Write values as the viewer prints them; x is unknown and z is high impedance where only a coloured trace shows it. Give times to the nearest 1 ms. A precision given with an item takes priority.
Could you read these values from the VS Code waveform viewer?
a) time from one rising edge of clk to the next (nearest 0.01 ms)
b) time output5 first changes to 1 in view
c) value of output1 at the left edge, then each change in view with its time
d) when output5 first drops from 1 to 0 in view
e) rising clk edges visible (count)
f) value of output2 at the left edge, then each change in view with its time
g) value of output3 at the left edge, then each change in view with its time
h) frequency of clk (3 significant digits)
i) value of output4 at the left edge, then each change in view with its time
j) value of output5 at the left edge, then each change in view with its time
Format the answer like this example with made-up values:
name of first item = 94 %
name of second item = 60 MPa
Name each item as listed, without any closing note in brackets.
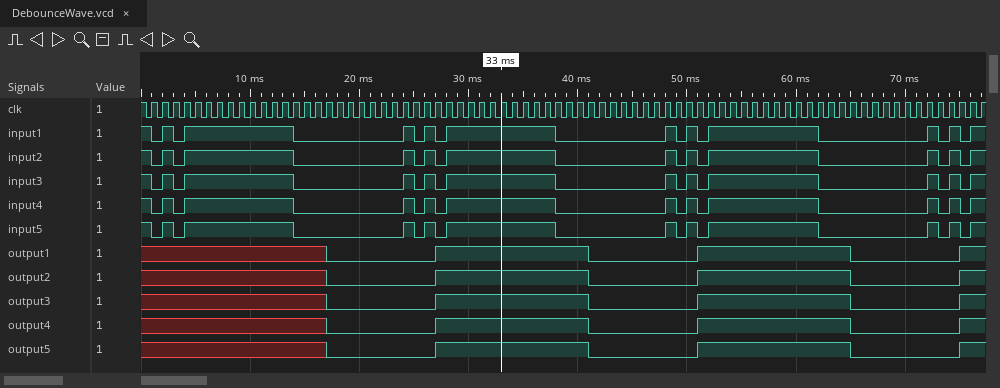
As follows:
time from one rising edge of clk to the next = 1 ms
time output5 first changes to 1 in view = 27 ms
value of output1 at the left edge, then each change in view with its time = x, 0 at 17 ms, 1 at 27 ms, 0 at 41 ms, 1 at 51 ms, 0 at 65 ms, 1 at 75 ms
when output5 first drops from 1 to 0 in view = 41 ms
rising clk edges visible = 77
value of output2 at the left edge, then each change in view with its time = x, 0 at 17 ms, 1 at 27 ms, 0 at 41 ms, 1 at 51 ms, 0 at 65 ms, 1 at 75 ms
value of output3 at the left edge, then each change in view with its time = x, 0 at 17 ms, 1 at 27 ms, 0 at 41 ms, 1 at 51 ms, 0 at 65 ms, 1 at 75 ms
frequency of clk = 1.00 kHz
value of output4 at the left edge, then each change in view with its time = x, 0 at 17 ms, 1 at 27 ms, 0 at 41 ms, 1 at 51 ms, 0 at 65 ms, 1 at 75 ms
value of output5 at the left edge, then each change in view with its time = x, 0 at 17 ms, 1 at 27 ms, 0 at 41 ms, 1 at 51 ms, 0 at 65 ms, 1 at 75 ms
